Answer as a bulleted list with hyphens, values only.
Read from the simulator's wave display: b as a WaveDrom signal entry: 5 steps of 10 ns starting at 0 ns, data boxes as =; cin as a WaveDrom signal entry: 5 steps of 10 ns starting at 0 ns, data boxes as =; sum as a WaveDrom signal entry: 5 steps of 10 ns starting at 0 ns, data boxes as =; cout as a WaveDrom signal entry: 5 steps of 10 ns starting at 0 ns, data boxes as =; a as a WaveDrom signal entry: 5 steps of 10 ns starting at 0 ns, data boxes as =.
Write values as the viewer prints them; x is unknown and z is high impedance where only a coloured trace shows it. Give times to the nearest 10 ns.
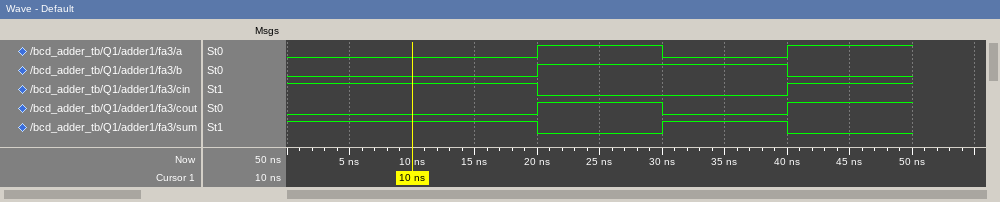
- {name: 'b', wave: '0.1.0'}
- {name: 'cin', wave: '1.0.1'}
- {name: 'sum', wave: '1.010'}
- {name: 'cout', wave: '0.101'}
- {name: 'a', wave: '0.101'}
